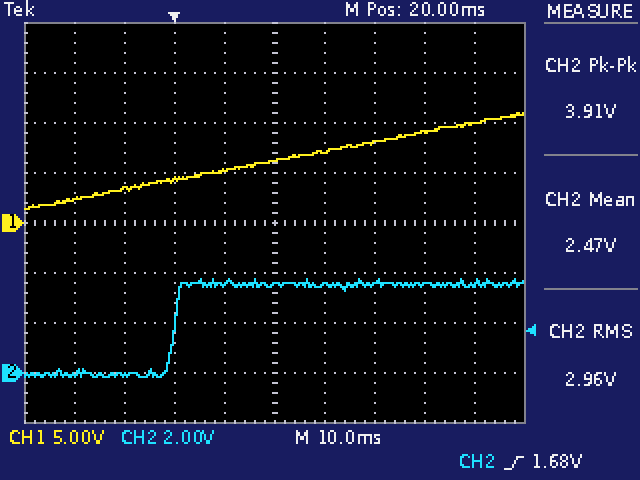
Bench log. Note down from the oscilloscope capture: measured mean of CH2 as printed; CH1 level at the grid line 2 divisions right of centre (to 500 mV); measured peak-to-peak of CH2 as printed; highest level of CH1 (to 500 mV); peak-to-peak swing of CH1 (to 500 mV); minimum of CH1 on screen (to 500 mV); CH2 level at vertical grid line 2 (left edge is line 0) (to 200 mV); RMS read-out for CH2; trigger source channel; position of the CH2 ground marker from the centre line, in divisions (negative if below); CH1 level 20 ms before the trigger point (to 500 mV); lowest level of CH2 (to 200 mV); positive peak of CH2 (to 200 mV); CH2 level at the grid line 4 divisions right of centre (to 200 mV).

2.47 V
8.0 V
3.91 V
11.0 V
9.5 V
1.5 V
0.0 V
2.96 V
CH2
-3.0 div
2.5 V
-200 mV
3.8 V
3.6 V
